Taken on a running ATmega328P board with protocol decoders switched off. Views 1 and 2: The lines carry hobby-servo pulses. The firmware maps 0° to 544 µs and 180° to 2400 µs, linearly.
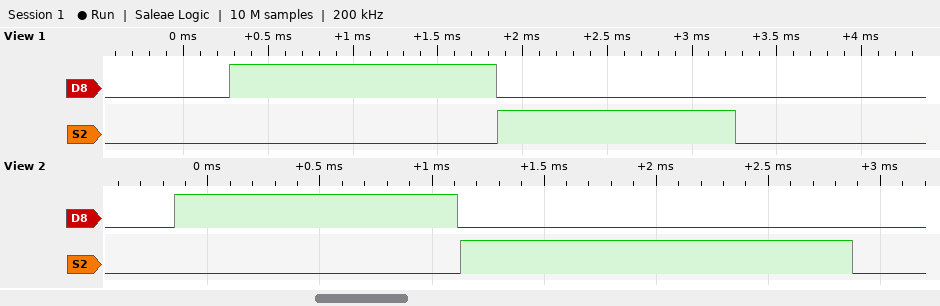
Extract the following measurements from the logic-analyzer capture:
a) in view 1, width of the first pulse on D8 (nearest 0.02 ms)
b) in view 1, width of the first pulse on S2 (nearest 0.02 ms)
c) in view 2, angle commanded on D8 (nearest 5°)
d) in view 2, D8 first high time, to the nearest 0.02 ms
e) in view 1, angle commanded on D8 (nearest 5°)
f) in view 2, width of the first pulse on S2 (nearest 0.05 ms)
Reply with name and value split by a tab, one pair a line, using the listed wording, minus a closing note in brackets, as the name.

in view 1, width of the first pulse on D8	1.58 ms
in view 1, width of the first pulse on S2	1.40 ms
in view 2, angle commanded on D8	70°
in view 2, D8 first high time, to the nearest 0.02 ms	1.26 ms
in view 1, angle commanded on D8	100°
in view 2, width of the first pulse on S2	1.75 ms
